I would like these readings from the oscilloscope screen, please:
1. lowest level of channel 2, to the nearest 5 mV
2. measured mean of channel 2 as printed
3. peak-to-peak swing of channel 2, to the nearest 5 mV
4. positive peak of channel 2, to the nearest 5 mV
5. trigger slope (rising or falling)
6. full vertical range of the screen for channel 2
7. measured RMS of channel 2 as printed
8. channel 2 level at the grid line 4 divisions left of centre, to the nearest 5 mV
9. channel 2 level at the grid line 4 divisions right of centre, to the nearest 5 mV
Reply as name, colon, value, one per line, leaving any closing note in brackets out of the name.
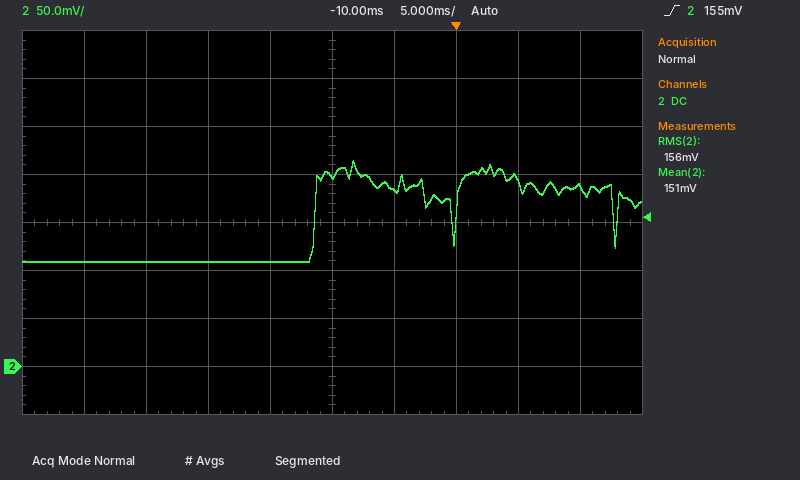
lowest level of channel 2, to the nearest 5 mV: 110 mV
measured mean of channel 2 as printed: 151 mV
peak-to-peak swing of channel 2, to the nearest 5 mV: 105 mV
positive peak of channel 2, to the nearest 5 mV: 215 mV
trigger slope: rising
full vertical range of the screen for channel 2: 400 mV
measured RMS of channel 2 as printed: 156 mV
channel 2 level at the grid line 4 divisions left of centre, to the nearest 5 mV: 110 mV
channel 2 level at the grid line 4 divisions right of centre, to the nearest 5 mV: 185 mV
